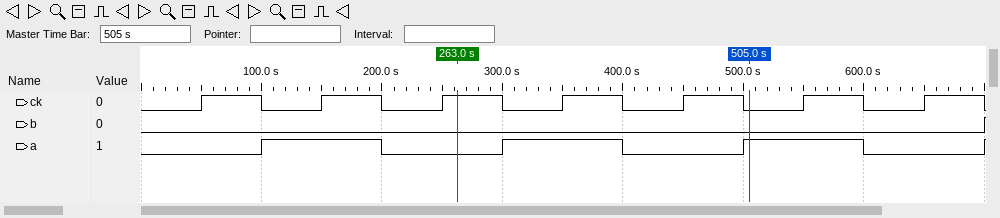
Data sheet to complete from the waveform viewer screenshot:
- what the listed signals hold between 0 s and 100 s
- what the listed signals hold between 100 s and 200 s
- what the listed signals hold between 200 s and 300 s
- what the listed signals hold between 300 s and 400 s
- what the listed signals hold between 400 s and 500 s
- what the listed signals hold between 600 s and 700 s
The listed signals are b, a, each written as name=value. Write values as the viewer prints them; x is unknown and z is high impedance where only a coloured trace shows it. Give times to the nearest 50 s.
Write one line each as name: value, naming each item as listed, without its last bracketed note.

what the listed signals hold between 0 s and 100 s: b=0, a=0
what the listed signals hold between 100 s and 200 s: b=0, a=1
what the listed signals hold between 200 s and 300 s: b=0, a=0
what the listed signals hold between 300 s and 400 s: b=0, a=1
what the listed signals hold between 400 s and 500 s: b=0, a=0
what the listed signals hold between 600 s and 700 s: b=0, a=0
